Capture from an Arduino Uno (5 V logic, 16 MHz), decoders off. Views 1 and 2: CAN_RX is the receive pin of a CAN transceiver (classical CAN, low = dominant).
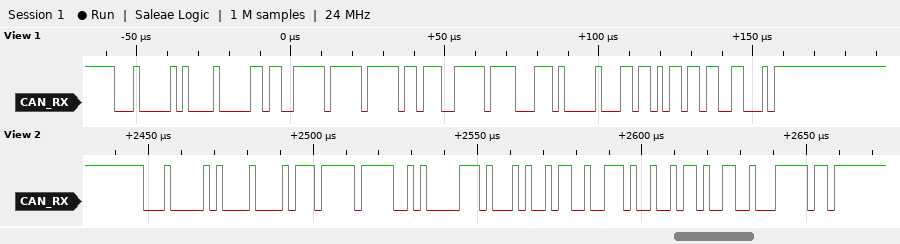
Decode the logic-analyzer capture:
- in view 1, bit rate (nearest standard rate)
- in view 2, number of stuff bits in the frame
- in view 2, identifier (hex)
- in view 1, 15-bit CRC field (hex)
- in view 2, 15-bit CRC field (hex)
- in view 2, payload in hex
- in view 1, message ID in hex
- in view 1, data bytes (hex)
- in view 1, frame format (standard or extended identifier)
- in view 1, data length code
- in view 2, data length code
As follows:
500 kbit/s
5
0x102
0x6D98
0x323F
5D FF A8 34 52 C9 D2 5A
0x102
2C FF FF B9 FF 1D 00 DA
standard
8
8
